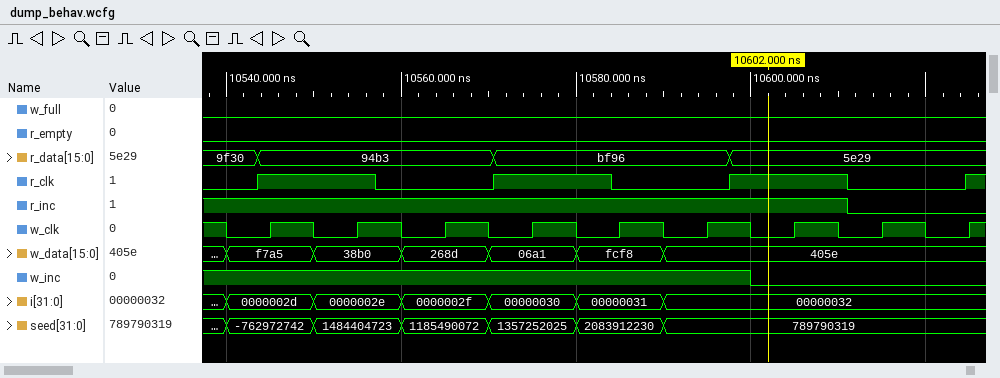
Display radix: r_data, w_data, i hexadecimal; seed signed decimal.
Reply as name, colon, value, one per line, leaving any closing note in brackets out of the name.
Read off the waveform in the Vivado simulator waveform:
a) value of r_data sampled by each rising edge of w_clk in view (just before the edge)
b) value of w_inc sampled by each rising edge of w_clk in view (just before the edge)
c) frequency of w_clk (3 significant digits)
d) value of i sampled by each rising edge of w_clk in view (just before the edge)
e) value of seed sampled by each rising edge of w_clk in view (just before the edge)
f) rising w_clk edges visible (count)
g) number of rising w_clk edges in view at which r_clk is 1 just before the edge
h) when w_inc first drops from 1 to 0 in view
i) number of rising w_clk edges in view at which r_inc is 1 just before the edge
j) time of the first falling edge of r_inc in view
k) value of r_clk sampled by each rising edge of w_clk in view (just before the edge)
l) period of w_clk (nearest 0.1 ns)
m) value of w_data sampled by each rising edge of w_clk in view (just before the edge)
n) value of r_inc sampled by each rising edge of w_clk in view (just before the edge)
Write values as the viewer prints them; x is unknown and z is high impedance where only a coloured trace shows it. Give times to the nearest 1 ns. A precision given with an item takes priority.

value of r_data sampled by each rising edge of w_clk in view: 94b3, 94b3, 94b3, bf96, bf96, bf96, 5e29, 5e29, 5e29
value of w_inc sampled by each rising edge of w_clk in view: 1 1 1 1 1 1 0 0 0
frequency of w_clk: 100 MHz
value of i sampled by each rising edge of w_clk in view: 0000002d, 0000002e, 0000002f, 00000030, 00000031, 00000032, 00000032, 00000032, 00000032
value of seed sampled by each rising edge of w_clk in view: -762972742, 1484404723, 1185490072, 1357252025, 2083912230, 789790319, 789790319, 789790319, 789790319
rising w_clk edges visible: 9
number of rising w_clk edges in view at which r_clk is 1 just before the edge: 5
when w_inc first drops from 1 to 0 in view: 10600 ns
number of rising w_clk edges in view at which r_inc is 1 just before the edge: 7
time of the first falling edge of r_inc in view: 10611 ns
value of r_clk sampled by each rising edge of w_clk in view: 1 1 0 1 0 0 1 0 1
period of w_clk: 10 ns
value of w_data sampled by each rising edge of w_clk in view: f7a5, 38b0, 268d, 06a1, fcf8, 405e, 405e, 405e, 405e
value of r_inc sampled by each rising edge of w_clk in view: 1 1 1 1 1 1 1 0 0
